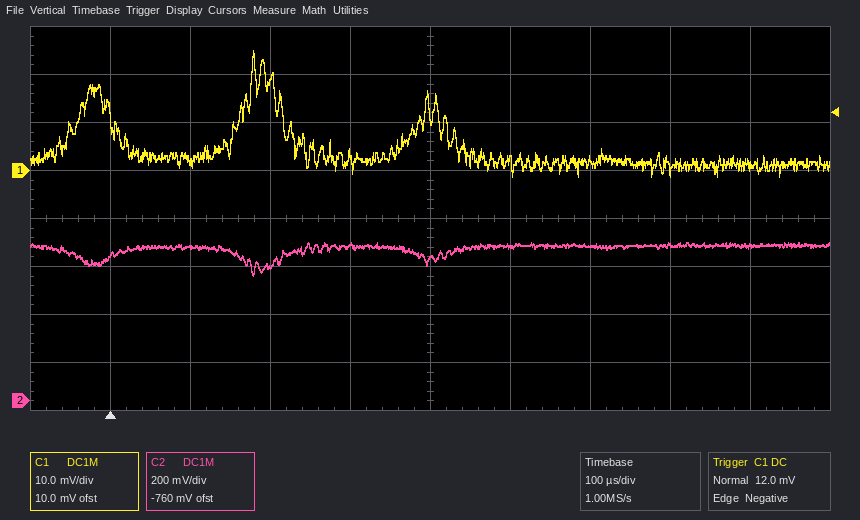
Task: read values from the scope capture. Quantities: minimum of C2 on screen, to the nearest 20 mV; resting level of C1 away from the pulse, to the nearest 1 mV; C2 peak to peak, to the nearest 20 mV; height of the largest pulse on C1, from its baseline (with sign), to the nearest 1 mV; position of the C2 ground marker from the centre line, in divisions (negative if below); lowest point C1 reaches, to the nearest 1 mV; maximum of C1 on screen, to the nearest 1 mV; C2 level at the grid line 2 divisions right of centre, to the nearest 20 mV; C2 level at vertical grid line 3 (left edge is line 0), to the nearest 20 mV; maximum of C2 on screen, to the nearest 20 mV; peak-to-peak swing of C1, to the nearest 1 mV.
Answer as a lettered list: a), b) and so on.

a) 520 mV
b) 2 mV
c) 140 mV
d) +23 mV
e) -3.8 div
f) -1 mV
g) 25 mV
h) 640 mV
i) 560 mV
j) 660 mV
k) 26 mV
